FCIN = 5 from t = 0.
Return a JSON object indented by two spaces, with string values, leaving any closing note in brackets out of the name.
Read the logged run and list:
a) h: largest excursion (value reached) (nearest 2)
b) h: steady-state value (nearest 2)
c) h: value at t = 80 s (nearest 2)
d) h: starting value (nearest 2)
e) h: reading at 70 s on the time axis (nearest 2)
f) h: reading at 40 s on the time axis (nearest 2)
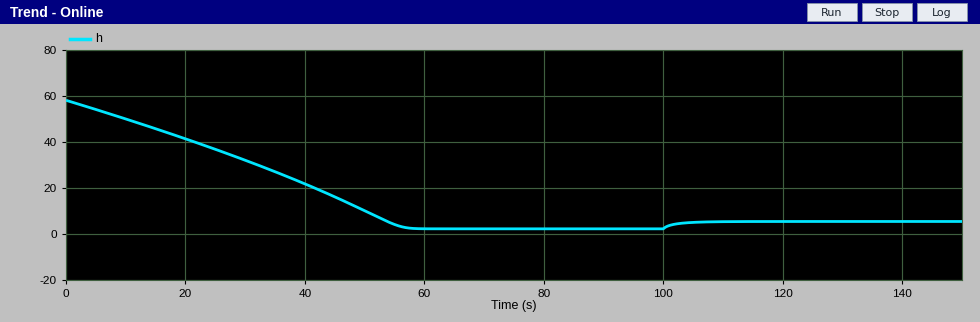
{
  "h: largest excursion (value reached)": "2",
  "h: steady-state value": "6",
  "h: value at t = 80 s": "2",
  "h: starting value": "58",
  "h: reading at 70 s on the time axis": "2",
  "h: reading at 40 s on the time axis": "22"
}
